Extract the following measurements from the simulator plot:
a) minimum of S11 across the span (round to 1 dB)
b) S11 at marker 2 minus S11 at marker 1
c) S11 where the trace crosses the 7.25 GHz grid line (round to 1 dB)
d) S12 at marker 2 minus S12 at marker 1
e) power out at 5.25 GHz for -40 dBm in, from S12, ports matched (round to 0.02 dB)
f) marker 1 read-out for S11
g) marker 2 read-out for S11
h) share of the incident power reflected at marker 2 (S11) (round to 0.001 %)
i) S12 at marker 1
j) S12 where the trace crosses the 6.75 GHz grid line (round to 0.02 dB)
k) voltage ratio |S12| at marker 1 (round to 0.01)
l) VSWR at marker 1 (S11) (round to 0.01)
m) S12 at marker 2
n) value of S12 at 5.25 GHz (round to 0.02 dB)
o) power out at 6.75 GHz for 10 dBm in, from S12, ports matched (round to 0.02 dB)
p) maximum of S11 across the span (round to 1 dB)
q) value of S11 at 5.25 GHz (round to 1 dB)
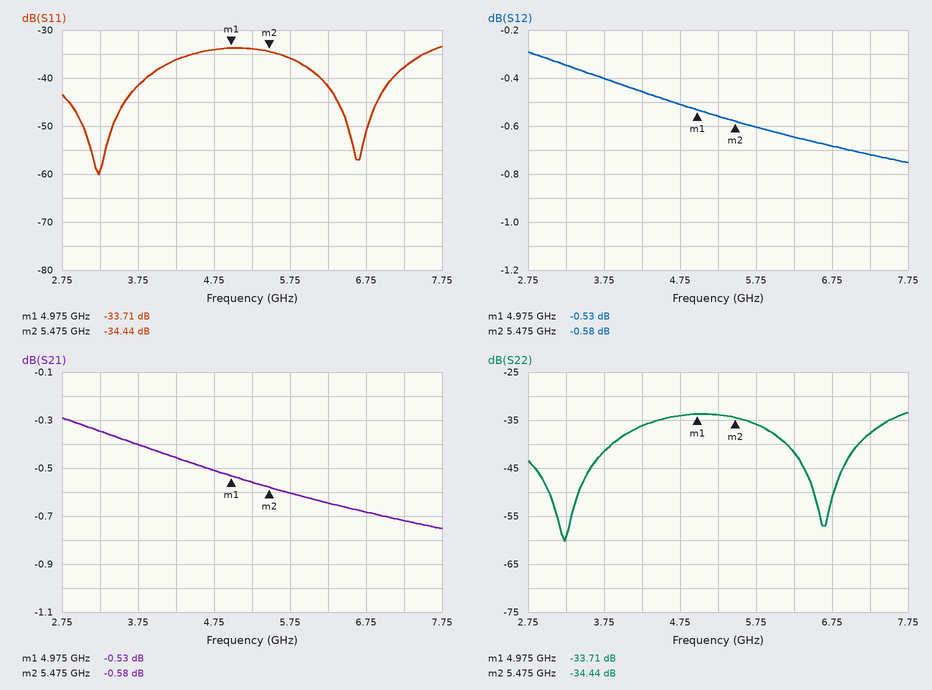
-60 dB
-0.73 dB
-38 dB
-0.05 dB
-40.56 dBm
-33.71 dB
-34.44 dB
0.036 %
-0.53 dB
-0.68 dB
0.94
1.04
-0.58 dB
-0.56 dB
9.32 dBm
-33 dB
-34 dB
